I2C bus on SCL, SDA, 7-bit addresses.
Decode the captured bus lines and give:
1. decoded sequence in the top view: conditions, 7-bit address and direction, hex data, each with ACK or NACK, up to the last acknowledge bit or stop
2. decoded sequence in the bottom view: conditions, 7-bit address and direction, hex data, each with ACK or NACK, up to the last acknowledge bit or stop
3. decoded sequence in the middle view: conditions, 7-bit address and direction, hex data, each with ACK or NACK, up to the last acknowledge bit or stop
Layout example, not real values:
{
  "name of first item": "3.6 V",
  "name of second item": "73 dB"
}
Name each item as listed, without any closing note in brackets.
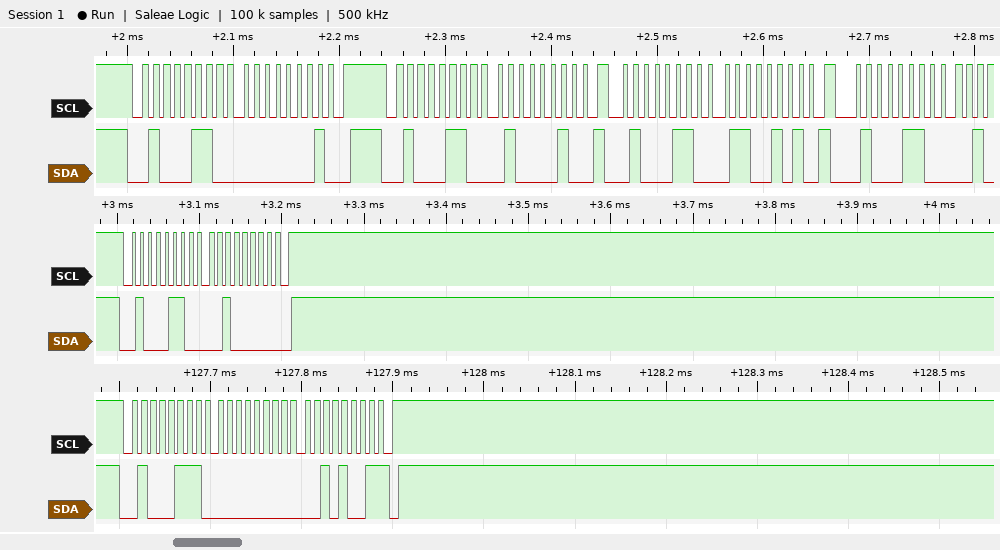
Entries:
{
  "decoded sequence in the top view: conditions, 7-bit address and direction, hex data, each with ACK or NACK, up to the last acknowledge bit or stop": "start, address 23 write ACK, 01 ACK, stop, start, address 23 write ACK, 42 ACK, repeated start, address 23 write ACK, 65 ACK, repeated start, address 23 write ACK",
  "decoded sequence in the bottom view: conditions, 7-bit address and direction, hex data, each with ACK or NACK, up to the last acknowledge bit or stop": "start, address 23 read ACK, 00 ACK, 29 NACK, stop",
  "decoded sequence in the middle view: conditions, 7-bit address and direction, hex data, each with ACK or NACK, up to the last acknowledge bit or stop": "start, address 23 write ACK, 20 ACK, stop"
}
